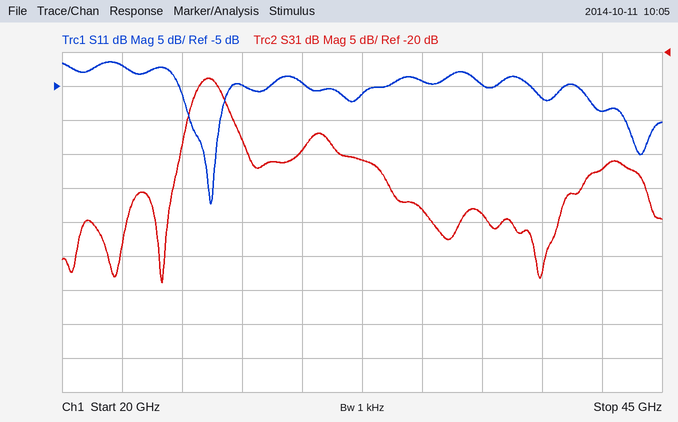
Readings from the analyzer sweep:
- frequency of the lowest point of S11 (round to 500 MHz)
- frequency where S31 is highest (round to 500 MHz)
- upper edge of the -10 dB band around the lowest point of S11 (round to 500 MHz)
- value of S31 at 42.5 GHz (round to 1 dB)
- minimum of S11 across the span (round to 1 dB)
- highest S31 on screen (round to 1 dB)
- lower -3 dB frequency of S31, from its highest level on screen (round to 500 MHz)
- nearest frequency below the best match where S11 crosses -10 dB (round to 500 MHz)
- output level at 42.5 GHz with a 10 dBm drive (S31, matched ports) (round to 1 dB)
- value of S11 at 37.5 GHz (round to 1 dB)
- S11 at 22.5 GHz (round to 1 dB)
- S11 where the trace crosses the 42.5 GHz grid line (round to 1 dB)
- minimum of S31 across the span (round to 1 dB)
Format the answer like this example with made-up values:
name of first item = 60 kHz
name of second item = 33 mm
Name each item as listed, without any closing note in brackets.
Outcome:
frequency of the lowest point of S11 = 26.0 GHz
frequency where S31 is highest = 26.0 GHz
upper edge of the -10 dB band around the lowest point of S11 = 26.5 GHz
value of S31 at 42.5 GHz = -37 dB
minimum of S11 across the span = -22 dB
highest S31 on screen = -24 dB
lower -3 dB frequency of S31, from its highest level on screen = 25.5 GHz
nearest frequency below the best match where S11 crosses -10 dB = 25.5 GHz
output level at 42.5 GHz with a 10 dBm drive (S31, matched ports) = -27 dBm
value of S11 at 37.5 GHz = -5 dB
S11 at 22.5 GHz = -2 dB
S11 where the trace crosses the 42.5 GHz grid line = -9 dB
minimum of S31 across the span = -54 dB
